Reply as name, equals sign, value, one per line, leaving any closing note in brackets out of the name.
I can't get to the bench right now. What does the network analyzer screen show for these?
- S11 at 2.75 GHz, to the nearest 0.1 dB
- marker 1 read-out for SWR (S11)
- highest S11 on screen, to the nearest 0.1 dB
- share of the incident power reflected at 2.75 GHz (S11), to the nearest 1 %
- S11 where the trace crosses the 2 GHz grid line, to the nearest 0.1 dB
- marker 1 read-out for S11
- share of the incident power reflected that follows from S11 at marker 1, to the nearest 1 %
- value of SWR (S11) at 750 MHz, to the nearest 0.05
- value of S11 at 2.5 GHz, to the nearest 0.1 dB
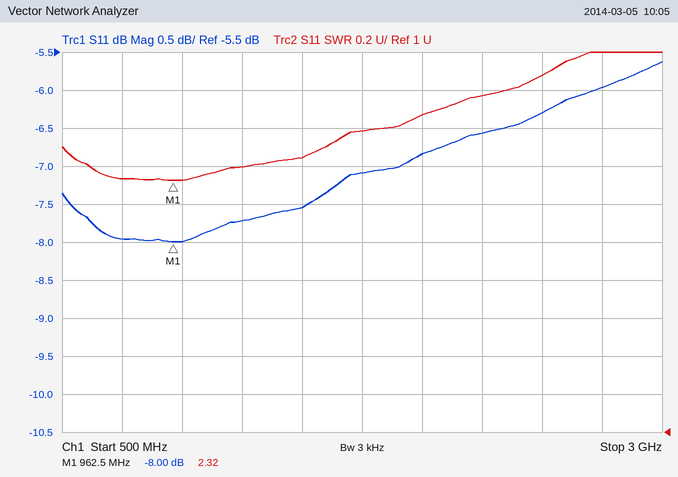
S11 at 2.75 GHz, to the nearest 0.1 dB = -6.0 dB
marker 1 read-out for SWR = 2.32
highest S11 on screen, to the nearest 0.1 dB = -5.6 dB
share of the incident power reflected at 2.75 GHz (S11), to the nearest 1 % = 25 %
S11 where the trace crosses the 2 GHz grid line, to the nearest 0.1 dB = -6.8 dB
marker 1 read-out for S11 = -8.00 dB
share of the incident power reflected that follows from S11 at marker 1, to the nearest 1 % = 16 %
value of SWR (S11) at 750 MHz, to the nearest 0.05 = 2.35
value of S11 at 2.5 GHz, to the nearest 0.1 dB = -6.3 dB
